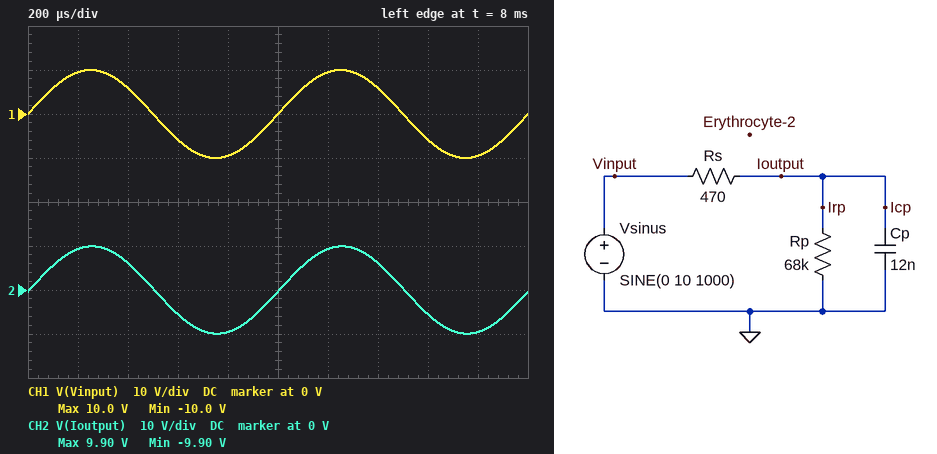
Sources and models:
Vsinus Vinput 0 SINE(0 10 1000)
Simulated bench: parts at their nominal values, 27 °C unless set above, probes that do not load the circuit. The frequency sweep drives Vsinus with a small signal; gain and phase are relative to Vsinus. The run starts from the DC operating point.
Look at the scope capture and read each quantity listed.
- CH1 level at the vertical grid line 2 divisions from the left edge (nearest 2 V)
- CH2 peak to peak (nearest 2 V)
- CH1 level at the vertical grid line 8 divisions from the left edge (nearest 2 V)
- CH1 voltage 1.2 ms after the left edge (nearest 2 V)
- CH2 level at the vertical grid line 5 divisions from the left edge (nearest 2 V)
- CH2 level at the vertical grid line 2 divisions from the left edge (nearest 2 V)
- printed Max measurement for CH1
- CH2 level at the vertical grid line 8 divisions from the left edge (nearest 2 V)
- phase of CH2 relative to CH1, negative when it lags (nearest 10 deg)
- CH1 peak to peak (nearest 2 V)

6 V
20 V
-6 V
10 V
0 V
6 V
10.0 V
-6 V
0 deg
20 V
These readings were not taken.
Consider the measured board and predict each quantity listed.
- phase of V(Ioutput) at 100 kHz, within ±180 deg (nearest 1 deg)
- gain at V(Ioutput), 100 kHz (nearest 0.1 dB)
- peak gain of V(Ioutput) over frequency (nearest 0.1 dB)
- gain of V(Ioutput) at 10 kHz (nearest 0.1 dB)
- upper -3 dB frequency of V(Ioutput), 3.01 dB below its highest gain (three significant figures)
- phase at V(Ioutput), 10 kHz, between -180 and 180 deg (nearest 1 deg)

-74 deg
-11.3 dB
-0.1 dB
-0.6 dB
28.4 kHz
-19 deg
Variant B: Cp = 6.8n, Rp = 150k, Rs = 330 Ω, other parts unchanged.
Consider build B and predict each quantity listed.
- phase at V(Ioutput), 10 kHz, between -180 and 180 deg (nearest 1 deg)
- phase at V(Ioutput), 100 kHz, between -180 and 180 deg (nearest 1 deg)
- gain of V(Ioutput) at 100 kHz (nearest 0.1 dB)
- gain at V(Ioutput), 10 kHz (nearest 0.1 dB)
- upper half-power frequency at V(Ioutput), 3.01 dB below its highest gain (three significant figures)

-8 deg
-55 deg
-4.8 dB
-0.1 dB
71.1 kHz
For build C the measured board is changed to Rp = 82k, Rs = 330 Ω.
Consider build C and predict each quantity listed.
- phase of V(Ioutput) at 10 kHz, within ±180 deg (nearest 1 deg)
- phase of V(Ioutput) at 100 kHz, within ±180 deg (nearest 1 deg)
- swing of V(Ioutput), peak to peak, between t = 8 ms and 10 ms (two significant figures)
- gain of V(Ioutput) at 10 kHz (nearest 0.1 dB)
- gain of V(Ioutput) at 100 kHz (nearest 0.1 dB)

-14 deg
-68 deg
20 V
-0.3 dB
-8.6 dB
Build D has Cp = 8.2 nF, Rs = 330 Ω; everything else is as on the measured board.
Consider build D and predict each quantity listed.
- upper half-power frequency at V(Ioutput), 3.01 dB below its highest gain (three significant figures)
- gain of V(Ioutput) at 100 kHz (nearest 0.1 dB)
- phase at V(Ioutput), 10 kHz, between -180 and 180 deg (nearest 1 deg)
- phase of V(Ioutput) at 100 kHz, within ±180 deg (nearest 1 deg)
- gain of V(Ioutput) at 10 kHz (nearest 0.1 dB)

59.1 kHz
-5.9 dB
-10 deg
-59 deg
-0.2 dB
